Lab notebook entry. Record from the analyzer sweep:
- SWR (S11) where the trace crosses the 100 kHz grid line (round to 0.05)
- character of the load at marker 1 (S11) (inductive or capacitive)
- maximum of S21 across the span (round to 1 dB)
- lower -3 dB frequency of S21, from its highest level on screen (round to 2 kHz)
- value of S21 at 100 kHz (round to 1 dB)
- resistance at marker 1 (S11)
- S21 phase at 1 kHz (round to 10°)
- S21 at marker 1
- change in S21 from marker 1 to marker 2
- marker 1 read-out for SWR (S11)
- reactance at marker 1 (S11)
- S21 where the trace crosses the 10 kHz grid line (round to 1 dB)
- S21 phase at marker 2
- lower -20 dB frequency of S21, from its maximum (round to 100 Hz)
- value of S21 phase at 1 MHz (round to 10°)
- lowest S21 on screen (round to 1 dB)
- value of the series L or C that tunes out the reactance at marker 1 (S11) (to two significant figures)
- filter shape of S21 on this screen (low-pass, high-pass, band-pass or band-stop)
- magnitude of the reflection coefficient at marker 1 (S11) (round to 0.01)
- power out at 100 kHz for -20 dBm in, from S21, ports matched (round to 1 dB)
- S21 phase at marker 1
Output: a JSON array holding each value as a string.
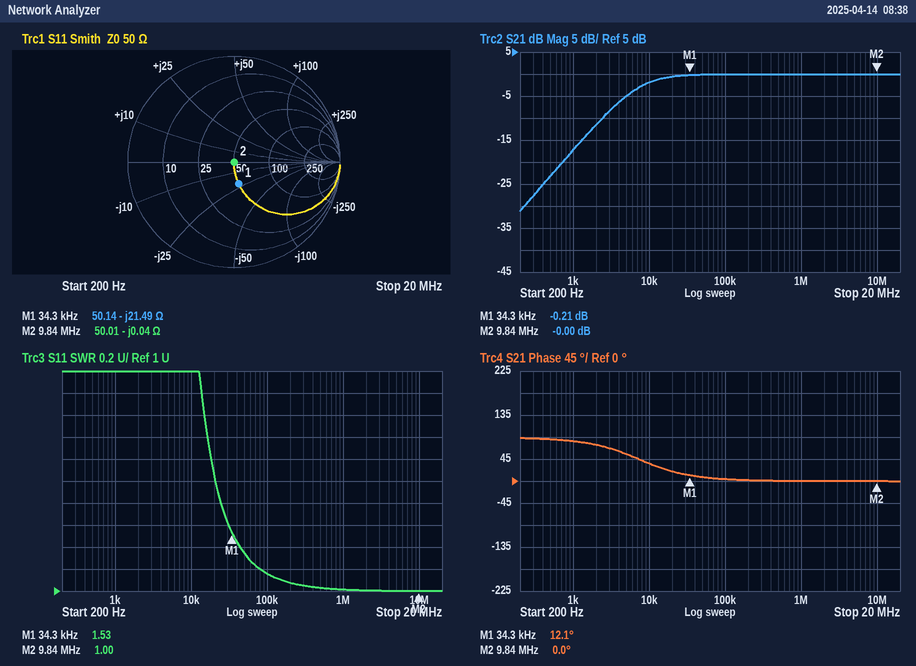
["1.15", "capacitive", "0 dB", "8 kHz", "0 dB", "50.14 Ω", "80°", "-0.21 dB", "0.21 dB", "1.53", "-21.49 Ω", "-2 dB", "0.0°", "700 Hz", "0°", "-31 dB", "100 µH", "high-pass", "0.21", "-20 dBm", "12.1°"]
